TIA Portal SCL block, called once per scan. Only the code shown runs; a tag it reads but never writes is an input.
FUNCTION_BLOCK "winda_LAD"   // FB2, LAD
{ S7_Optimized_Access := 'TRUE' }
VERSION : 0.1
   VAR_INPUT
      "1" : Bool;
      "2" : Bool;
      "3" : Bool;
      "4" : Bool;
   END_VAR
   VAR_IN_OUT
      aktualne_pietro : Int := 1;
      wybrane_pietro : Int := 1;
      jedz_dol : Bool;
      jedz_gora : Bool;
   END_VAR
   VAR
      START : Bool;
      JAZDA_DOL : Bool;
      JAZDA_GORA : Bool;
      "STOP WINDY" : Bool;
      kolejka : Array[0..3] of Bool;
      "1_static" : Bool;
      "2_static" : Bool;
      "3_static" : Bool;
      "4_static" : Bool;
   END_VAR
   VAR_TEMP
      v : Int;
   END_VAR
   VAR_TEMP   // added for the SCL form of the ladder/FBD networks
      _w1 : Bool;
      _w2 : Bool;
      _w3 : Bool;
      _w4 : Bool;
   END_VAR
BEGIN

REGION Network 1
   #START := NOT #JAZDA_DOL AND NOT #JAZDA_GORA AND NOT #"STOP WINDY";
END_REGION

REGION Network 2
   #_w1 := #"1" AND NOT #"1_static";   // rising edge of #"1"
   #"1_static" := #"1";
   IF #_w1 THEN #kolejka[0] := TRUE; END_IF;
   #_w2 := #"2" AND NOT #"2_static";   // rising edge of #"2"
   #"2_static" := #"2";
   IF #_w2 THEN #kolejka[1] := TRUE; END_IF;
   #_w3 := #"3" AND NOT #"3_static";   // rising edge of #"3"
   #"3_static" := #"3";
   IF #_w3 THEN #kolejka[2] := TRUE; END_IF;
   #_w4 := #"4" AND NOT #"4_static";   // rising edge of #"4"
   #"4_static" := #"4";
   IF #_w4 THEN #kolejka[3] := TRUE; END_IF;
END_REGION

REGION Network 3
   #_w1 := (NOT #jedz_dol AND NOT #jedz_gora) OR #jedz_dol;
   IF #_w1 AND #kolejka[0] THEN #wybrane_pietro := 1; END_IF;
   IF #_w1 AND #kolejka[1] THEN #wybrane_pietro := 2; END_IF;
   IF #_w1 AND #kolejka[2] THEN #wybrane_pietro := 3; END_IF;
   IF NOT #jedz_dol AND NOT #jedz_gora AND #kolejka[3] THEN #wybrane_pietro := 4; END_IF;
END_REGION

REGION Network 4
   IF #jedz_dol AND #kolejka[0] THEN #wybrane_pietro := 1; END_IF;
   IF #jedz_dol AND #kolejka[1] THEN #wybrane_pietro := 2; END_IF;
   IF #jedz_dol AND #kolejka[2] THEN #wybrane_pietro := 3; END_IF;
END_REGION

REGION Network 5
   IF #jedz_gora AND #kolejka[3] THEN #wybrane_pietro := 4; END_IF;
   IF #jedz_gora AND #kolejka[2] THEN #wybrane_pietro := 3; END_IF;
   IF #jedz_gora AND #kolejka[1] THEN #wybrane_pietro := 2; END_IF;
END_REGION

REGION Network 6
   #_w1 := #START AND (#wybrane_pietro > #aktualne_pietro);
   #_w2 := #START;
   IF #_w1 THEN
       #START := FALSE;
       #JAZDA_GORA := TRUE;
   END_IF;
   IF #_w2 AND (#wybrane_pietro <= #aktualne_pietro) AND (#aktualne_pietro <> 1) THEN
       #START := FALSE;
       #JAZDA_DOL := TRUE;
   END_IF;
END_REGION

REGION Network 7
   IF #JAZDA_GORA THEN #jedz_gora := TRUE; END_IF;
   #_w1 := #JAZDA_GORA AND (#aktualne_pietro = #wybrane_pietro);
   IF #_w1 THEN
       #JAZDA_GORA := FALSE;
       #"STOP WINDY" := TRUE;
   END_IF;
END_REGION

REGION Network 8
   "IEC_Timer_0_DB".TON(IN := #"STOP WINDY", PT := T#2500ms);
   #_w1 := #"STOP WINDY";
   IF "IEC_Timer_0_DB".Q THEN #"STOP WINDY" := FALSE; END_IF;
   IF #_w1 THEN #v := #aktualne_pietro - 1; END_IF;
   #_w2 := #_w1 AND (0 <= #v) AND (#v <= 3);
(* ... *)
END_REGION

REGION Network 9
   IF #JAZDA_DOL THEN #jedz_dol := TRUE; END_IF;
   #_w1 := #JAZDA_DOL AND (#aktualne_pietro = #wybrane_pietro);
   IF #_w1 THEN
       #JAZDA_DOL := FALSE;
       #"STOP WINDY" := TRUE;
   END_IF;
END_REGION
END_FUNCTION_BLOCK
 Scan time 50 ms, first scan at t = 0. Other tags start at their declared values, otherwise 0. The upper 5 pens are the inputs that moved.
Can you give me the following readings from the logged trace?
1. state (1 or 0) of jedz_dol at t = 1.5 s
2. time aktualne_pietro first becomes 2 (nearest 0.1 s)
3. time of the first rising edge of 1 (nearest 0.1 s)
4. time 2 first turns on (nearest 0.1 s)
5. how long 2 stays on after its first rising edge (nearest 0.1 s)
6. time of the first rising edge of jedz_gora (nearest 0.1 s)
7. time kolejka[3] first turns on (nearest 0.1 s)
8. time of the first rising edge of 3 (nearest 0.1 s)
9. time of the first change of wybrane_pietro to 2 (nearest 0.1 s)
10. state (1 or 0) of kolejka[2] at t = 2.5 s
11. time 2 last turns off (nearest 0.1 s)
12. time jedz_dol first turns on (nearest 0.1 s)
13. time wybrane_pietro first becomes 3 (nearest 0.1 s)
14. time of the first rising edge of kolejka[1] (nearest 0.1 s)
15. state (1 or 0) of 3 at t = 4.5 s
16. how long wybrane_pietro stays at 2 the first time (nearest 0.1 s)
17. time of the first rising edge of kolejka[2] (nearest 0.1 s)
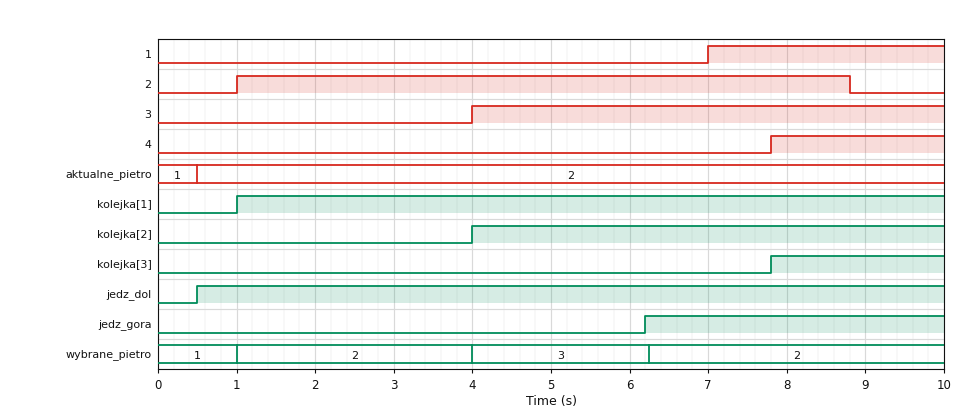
1
0.5 s
7.0 s
1.0 s
7.8 s
6.2 s
7.8 s
4.0 s
1.0 s
0
8.8 s
0.5 s
4.0 s
1.0 s
1
3.0 s
4.0 s
